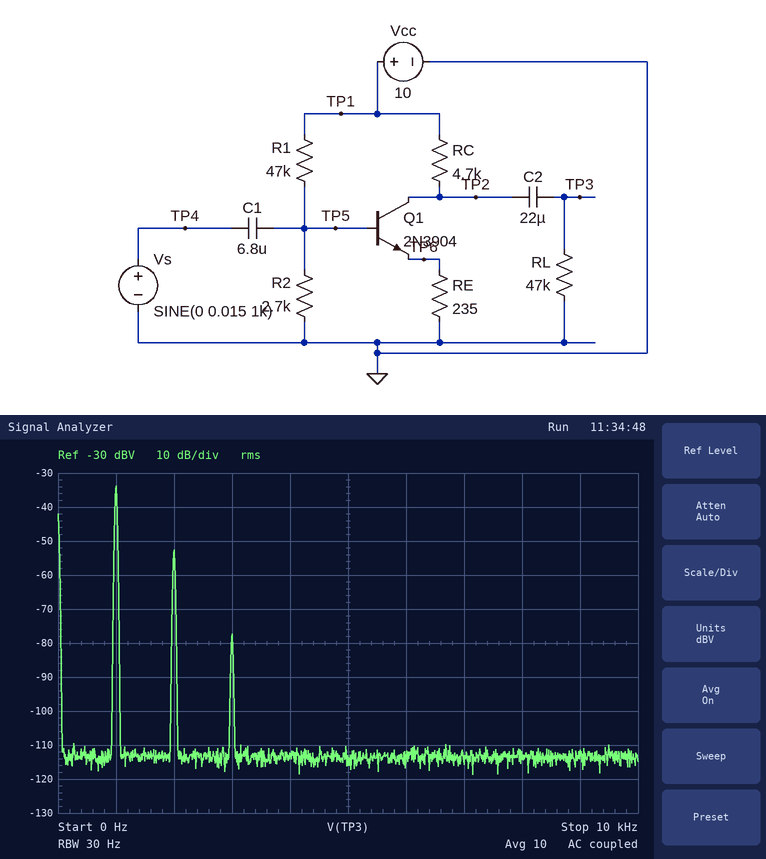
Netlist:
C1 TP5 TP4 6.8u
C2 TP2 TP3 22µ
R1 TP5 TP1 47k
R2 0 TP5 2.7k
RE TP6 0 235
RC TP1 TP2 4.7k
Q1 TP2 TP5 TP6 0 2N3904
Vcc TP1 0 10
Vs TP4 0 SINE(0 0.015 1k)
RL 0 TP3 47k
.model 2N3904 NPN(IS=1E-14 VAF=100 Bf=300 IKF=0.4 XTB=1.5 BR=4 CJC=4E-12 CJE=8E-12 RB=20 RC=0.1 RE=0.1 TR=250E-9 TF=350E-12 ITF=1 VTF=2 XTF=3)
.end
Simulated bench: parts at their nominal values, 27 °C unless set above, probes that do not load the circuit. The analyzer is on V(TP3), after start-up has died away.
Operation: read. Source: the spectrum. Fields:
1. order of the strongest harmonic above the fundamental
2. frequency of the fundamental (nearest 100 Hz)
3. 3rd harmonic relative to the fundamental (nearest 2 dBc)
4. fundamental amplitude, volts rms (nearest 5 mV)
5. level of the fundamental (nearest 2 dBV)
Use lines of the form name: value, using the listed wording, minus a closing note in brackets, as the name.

order of the strongest harmonic above the fundamental: 2
frequency of the fundamental: 1.0 kHz
3rd harmonic relative to the fundamental: -44 dBc
fundamental amplitude, volts rms: 20 mV
level of the fundamental: -34 dBV
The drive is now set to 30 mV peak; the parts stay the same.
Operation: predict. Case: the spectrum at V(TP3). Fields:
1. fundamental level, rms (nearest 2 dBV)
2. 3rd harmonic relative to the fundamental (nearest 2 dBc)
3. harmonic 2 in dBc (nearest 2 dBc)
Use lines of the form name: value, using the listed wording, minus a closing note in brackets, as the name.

fundamental level, rms: -28 dBV
3rd harmonic relative to the fundamental: -32 dBc
harmonic 2 in dBc: -14 dBc
